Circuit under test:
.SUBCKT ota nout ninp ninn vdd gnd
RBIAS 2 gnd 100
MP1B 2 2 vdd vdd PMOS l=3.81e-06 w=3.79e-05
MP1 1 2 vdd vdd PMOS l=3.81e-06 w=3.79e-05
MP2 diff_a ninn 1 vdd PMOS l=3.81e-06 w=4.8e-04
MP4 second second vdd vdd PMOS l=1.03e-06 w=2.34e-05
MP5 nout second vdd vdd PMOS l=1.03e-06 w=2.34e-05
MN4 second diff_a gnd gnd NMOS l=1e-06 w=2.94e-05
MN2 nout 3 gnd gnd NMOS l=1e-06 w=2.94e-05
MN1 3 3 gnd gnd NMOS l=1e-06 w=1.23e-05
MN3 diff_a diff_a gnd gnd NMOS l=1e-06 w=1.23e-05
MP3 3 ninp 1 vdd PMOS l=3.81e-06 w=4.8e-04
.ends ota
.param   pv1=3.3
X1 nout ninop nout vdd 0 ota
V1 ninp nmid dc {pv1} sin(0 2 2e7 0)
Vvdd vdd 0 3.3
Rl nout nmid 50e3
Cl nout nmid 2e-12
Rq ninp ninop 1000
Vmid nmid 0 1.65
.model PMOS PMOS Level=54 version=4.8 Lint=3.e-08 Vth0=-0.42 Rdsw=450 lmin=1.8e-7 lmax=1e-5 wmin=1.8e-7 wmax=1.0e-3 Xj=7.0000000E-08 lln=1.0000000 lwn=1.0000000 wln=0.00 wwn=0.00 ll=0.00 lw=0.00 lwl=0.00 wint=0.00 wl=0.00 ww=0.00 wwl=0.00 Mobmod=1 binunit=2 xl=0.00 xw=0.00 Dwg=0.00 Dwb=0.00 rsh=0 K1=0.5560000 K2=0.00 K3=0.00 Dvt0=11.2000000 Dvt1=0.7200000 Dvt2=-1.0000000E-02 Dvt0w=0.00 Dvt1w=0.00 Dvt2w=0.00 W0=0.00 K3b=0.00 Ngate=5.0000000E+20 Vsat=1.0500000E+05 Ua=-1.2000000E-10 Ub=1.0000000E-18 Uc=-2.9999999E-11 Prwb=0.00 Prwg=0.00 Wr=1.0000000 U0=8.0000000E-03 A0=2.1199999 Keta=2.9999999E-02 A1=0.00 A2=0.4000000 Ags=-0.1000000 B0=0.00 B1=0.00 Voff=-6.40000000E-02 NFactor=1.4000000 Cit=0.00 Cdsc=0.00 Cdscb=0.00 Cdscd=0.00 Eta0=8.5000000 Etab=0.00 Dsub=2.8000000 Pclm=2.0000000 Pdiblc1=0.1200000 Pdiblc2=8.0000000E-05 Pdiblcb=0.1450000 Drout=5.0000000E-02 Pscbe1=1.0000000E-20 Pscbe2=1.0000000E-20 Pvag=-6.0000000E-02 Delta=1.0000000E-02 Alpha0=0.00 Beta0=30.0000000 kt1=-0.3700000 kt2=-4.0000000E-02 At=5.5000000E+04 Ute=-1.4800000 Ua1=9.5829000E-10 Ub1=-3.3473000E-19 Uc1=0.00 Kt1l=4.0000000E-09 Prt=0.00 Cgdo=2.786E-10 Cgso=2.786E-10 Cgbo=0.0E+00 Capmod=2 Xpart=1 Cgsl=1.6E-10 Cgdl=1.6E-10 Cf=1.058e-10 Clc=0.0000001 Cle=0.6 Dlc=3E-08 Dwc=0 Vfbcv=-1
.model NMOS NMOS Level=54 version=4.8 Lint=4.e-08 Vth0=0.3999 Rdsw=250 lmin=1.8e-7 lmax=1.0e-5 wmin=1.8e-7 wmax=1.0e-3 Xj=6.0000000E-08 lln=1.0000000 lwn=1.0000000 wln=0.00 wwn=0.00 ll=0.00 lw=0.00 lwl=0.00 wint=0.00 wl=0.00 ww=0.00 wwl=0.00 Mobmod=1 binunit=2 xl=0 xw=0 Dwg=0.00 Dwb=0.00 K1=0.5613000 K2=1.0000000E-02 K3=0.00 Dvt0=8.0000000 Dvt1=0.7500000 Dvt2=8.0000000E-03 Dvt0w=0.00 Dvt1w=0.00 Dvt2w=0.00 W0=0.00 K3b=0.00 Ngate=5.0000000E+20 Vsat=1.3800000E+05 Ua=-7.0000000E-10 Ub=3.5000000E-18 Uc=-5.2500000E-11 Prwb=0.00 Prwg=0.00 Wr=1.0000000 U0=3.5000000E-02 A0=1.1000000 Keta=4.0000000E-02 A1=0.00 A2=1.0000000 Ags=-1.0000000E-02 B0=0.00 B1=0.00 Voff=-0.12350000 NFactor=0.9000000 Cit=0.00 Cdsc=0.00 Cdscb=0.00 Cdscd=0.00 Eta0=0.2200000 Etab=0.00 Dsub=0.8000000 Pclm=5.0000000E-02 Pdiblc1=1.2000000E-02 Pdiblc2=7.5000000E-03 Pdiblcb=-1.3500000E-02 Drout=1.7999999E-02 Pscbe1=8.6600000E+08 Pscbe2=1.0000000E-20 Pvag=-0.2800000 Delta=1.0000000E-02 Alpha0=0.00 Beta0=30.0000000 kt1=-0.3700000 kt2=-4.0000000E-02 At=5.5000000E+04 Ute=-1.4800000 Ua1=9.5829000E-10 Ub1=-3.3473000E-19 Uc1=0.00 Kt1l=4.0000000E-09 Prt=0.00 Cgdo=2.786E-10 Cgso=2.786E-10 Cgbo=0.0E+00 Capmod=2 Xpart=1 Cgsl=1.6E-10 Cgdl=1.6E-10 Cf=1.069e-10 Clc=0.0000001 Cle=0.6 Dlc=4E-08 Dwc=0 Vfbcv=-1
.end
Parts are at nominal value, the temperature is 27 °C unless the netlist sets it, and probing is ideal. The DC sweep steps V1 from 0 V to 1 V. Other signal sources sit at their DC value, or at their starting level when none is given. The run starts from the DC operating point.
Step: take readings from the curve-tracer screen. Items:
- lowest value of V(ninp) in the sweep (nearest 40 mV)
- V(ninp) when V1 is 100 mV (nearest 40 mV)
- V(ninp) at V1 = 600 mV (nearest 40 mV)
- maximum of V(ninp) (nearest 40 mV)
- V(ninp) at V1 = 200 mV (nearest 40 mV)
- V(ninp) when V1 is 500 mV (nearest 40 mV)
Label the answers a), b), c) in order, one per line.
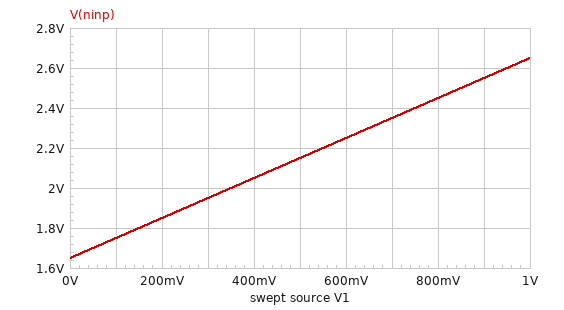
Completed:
a) 1.64 V
b) 1.76 V
c) 2.24 V
d) 2.64 V
e) 1.84 V
f) 2.16 V
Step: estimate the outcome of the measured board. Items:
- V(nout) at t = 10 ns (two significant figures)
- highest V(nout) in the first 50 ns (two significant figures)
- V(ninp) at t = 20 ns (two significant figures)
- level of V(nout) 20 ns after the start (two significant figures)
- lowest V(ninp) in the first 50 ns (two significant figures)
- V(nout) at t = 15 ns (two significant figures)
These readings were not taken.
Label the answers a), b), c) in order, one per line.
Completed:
a) 2.4 V
b) 2.8 V
c) 2.8 V
d) 2.8 V
e) -350 mV
f) 2.7 V
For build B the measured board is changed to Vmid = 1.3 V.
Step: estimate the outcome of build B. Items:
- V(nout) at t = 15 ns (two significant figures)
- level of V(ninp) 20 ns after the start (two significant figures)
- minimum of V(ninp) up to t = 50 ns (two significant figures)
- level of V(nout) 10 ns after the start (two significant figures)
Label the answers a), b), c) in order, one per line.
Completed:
a) 2.6 V
b) 2.5 V
c) -700 mV
d) 2.2 V
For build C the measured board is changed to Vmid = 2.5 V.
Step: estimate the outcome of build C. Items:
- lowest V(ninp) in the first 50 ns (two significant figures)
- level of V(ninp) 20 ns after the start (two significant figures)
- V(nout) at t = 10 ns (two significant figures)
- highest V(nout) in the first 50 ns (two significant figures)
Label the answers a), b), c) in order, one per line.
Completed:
a) 500 mV
b) 3.7 V
c) 2.8 V
d) 2.9 V
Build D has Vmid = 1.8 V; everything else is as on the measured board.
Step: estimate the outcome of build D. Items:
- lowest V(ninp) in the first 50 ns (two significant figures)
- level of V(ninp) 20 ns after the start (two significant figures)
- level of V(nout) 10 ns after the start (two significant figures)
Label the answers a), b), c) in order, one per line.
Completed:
a) -200 mV
b) 3.0 V
c) 2.5 V
